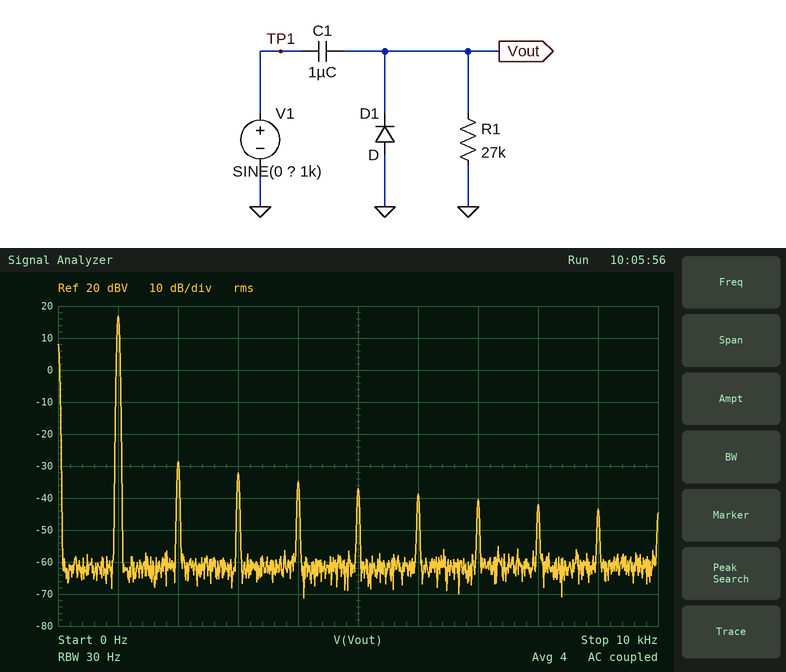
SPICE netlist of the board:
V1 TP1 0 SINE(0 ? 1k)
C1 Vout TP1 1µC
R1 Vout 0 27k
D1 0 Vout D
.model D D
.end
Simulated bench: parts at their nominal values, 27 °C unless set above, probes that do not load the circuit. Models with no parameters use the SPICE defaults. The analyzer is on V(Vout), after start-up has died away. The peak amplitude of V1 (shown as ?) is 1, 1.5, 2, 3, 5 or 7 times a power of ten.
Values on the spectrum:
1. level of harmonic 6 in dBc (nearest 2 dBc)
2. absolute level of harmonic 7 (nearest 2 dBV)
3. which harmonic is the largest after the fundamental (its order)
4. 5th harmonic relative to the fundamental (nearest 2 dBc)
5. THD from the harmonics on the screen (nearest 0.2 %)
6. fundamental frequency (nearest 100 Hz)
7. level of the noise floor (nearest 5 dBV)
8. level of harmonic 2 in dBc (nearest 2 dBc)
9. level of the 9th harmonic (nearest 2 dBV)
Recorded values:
-56 dBc
-40 dBV
2
-54 dBc
0.8 %
1.0 kHz
-60 dBV
-46 dBc
-44 dBV
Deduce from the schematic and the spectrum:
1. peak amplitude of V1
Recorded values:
10 V
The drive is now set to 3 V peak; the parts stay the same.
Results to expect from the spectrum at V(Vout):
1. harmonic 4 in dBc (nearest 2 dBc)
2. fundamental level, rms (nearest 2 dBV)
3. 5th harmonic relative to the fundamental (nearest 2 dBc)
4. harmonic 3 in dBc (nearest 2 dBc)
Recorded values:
-54 dBc
6 dBV
-56 dBc
-50 dBc
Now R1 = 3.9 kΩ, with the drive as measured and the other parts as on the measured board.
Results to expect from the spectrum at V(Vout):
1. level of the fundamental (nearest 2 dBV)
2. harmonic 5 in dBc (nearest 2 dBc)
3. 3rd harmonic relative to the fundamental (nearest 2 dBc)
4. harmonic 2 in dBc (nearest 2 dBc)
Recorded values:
16 dBV
-40 dBc
-34 dBc
-30 dBc
